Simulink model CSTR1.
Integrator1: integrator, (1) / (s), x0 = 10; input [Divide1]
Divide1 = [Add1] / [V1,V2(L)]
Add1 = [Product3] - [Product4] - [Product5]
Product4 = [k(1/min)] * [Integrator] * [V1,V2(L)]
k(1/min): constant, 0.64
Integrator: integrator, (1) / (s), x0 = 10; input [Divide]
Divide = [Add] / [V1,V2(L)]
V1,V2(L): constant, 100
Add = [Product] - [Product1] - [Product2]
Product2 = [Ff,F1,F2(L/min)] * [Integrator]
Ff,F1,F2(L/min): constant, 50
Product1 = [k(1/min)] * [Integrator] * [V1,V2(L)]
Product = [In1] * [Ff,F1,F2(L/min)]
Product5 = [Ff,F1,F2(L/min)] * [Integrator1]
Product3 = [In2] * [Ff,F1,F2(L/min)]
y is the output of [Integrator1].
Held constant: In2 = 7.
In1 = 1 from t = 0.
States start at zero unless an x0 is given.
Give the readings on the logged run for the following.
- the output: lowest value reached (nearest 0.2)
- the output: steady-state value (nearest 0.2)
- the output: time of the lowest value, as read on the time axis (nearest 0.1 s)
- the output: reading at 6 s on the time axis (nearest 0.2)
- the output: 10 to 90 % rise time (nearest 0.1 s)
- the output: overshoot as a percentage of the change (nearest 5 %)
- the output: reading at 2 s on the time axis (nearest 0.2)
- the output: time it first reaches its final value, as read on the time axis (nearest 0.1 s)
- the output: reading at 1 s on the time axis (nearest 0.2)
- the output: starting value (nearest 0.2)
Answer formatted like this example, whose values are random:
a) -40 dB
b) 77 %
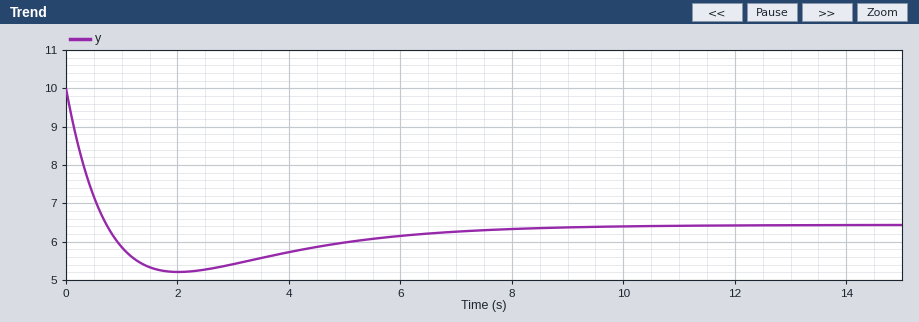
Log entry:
a) 5.2
b) 6.4
c) 2.0 s
d) 6.2
e) 0.6 s
f) 35 %
g) 5.2
h) 0.7 s
i) 5.8
j) 10.0
